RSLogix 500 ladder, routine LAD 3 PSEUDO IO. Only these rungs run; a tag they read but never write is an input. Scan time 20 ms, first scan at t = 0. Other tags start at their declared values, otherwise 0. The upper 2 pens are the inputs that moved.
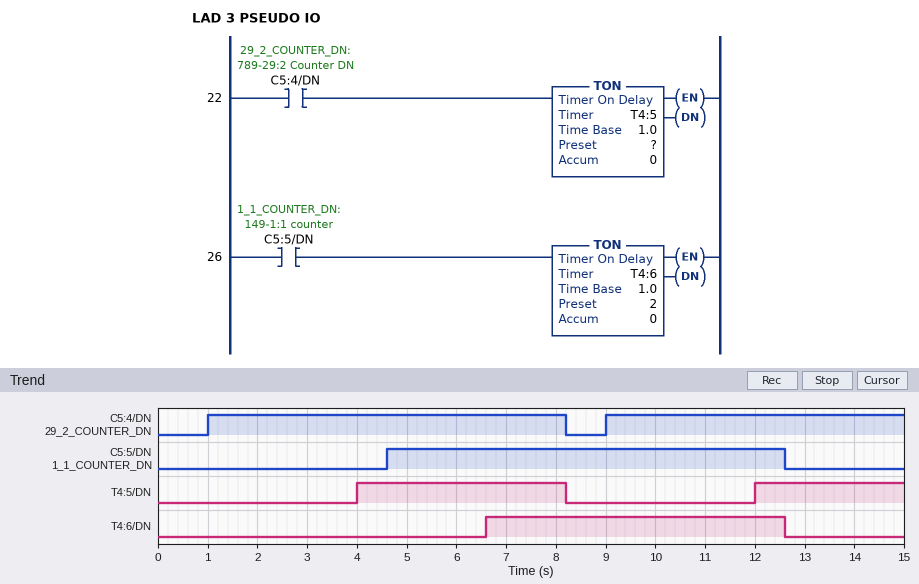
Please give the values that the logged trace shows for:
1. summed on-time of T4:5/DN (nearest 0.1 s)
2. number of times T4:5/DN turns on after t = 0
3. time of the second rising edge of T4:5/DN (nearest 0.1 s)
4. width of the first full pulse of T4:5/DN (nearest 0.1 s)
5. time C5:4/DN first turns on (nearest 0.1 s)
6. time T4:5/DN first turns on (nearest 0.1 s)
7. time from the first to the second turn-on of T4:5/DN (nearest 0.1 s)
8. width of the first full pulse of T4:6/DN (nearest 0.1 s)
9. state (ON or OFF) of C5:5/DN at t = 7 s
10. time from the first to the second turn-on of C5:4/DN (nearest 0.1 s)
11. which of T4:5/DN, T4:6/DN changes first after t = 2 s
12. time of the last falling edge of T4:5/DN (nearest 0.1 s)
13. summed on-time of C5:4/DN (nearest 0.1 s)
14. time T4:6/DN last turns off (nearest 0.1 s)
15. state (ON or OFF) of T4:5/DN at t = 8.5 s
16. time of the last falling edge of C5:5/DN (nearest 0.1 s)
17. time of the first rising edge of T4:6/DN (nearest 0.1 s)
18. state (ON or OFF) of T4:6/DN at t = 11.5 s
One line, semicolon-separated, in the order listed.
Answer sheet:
7.2 s; 2; 12.0 s; 4.2 s; 1.0 s; 4.0 s; 8.0 s; 6.0 s; ON; 8.0 s; T4:5/DN; 8.2 s; 13.2 s; 12.6 s; OFF; 12.6 s; 6.6 s; ON
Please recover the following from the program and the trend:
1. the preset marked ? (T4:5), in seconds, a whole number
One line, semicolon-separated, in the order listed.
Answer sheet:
3 s
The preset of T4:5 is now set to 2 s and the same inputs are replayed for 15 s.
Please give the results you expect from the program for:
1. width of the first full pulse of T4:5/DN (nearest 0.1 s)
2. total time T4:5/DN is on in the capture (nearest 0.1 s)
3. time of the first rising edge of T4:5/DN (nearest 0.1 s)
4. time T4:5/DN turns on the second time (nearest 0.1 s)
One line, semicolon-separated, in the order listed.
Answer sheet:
5.2 s; 9.2 s; 3.0 s; 11.0 s
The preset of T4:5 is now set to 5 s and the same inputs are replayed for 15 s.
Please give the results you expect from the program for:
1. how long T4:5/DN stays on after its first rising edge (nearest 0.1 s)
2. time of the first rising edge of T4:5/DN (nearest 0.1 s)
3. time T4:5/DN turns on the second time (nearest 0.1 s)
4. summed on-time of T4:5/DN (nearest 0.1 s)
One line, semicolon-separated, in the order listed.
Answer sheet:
2.2 s; 6.0 s; 14.0 s; 3.2 s
